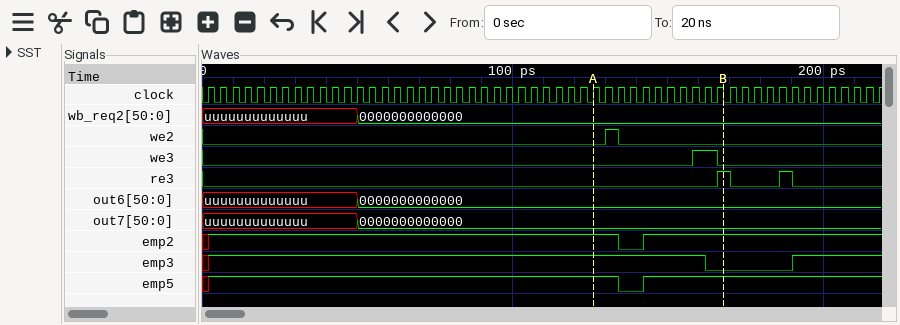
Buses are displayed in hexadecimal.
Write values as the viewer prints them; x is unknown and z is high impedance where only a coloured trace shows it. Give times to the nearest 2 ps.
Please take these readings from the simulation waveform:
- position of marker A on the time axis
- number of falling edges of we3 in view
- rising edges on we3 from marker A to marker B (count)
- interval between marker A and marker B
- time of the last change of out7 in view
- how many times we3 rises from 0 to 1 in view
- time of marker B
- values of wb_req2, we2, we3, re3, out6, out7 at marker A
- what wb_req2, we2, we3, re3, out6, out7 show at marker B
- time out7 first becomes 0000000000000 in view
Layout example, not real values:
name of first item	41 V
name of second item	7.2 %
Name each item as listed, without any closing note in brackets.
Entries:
position of marker A on the time axis	126 ps
number of falling edges of we3 in view	1
rising edges on we3 from marker A to marker B	1
interval between marker A and marker B	42 ps
time of the last change of out7 in view	50 ps
how many times we3 rises from 0 to 1 in view	1
time of marker B	168 ps
values of wb_req2, we2, we3, re3, out6, out7 at marker A	wb_req2=0000000000000, we2=0, we3=0, re3=0, out6=0000000000000, out7=0000000000000
what wb_req2, we2, we3, re3, out6, out7 show at marker B	wb_req2=0000000000000, we2=0, we3=0, re3=1, out6=0000000000000, out7=0000000000000
time out7 first becomes 0000000000000 in view	50 ps
